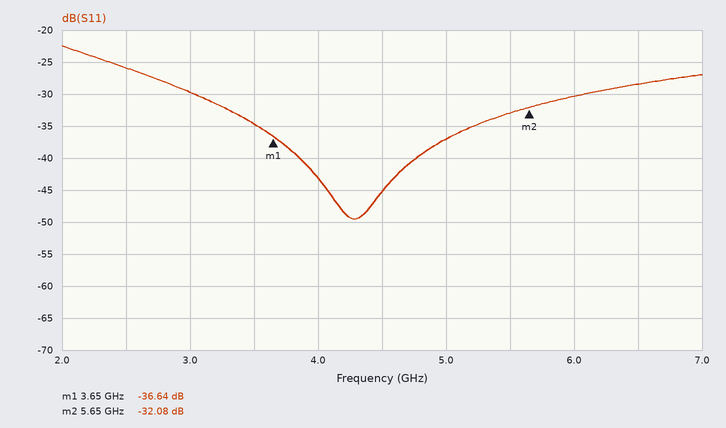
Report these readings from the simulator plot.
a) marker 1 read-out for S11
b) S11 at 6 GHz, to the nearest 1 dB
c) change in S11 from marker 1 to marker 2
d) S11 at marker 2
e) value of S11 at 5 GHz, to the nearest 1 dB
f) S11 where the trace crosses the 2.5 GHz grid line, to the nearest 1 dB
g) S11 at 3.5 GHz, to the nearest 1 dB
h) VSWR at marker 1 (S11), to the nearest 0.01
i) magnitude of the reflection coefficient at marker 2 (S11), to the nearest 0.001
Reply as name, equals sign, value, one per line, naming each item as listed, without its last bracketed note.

marker 1 read-out for S11 = -36.64 dB
S11 at 6 GHz, to the nearest 1 dB = -30 dB
change in S11 from marker 1 to marker 2 = 4.56 dB
S11 at marker 2 = -32.08 dB
value of S11 at 5 GHz, to the nearest 1 dB = -37 dB
S11 where the trace crosses the 2.5 GHz grid line, to the nearest 1 dB = -26 dB
S11 at 3.5 GHz, to the nearest 1 dB = -35 dB
VSWR at marker 1 (S11), to the nearest 0.01 = 1.03
magnitude of the reflection coefficient at marker 2 (S11), to the nearest 0.001 = 0.025
